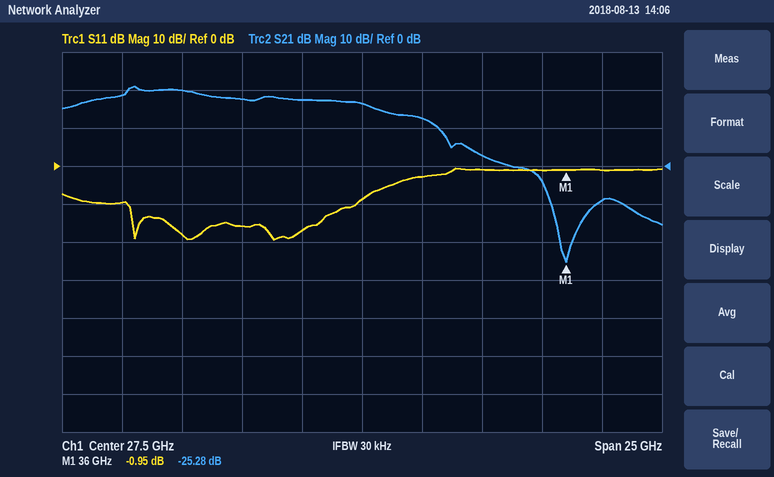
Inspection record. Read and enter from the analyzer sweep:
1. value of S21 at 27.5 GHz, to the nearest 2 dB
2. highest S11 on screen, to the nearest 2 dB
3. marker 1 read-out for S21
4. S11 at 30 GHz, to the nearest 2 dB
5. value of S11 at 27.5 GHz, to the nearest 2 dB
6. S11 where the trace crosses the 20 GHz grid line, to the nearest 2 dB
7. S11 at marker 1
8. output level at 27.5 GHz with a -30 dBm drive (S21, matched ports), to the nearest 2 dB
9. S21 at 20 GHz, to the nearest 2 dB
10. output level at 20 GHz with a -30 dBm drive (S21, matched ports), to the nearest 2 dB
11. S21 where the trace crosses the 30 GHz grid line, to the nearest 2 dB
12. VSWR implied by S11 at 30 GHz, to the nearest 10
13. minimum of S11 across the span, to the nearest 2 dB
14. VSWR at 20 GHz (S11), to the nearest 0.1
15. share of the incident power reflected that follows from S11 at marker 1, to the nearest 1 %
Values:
16 dB
0 dB
-25.28 dB
-2 dB
-8 dB
-18 dB
-0.95 dB
-14 dBm
20 dB
-10 dBm
12 dB
10
-20 dB
1.3
80 %
